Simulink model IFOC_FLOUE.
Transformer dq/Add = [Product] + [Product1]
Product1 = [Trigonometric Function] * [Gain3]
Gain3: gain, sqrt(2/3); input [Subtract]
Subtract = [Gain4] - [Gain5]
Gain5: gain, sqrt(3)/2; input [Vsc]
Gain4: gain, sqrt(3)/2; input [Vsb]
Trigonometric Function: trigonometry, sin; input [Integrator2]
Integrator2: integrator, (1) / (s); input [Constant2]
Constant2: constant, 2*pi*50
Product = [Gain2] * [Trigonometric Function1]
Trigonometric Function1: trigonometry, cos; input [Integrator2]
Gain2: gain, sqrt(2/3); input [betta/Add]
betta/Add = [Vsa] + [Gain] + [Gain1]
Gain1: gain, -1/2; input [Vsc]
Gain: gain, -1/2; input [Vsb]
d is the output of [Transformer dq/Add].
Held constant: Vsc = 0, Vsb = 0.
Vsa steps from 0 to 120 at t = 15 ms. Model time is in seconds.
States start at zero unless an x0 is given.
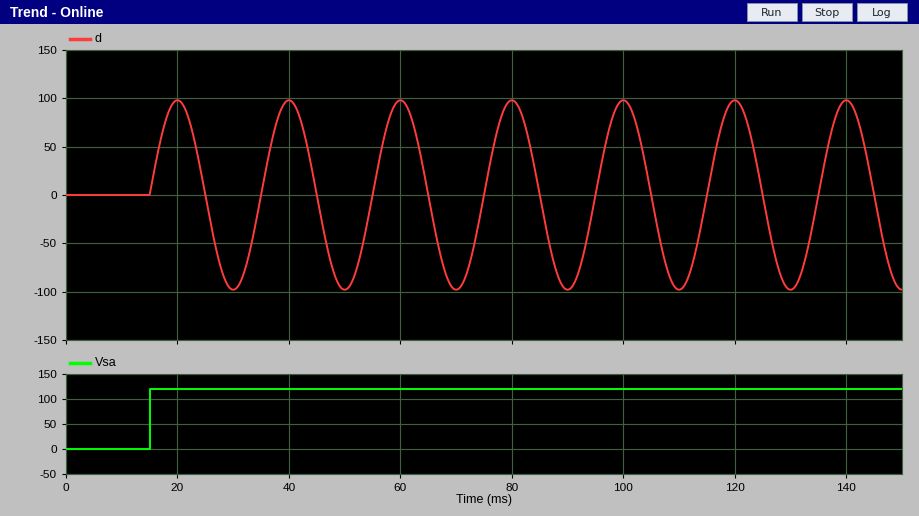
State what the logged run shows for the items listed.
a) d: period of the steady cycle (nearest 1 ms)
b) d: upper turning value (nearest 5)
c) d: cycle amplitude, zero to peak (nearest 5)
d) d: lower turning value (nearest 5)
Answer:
20 ms
100
100
-100
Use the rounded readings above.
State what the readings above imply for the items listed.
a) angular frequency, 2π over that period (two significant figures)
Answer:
0.31 rad/ms
